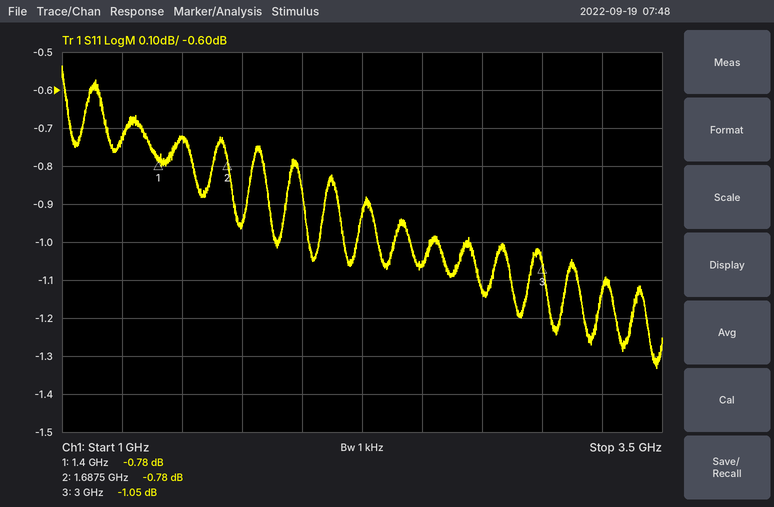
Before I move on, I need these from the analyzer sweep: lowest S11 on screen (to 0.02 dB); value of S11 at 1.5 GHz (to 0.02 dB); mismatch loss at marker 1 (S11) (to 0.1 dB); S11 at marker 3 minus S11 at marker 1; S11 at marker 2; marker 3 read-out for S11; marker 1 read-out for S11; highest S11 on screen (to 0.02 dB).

-1.34 dB
-0.72 dB
7.8 dB
-0.27 dB
-0.78 dB
-1.05 dB
-0.78 dB
-0.54 dB
